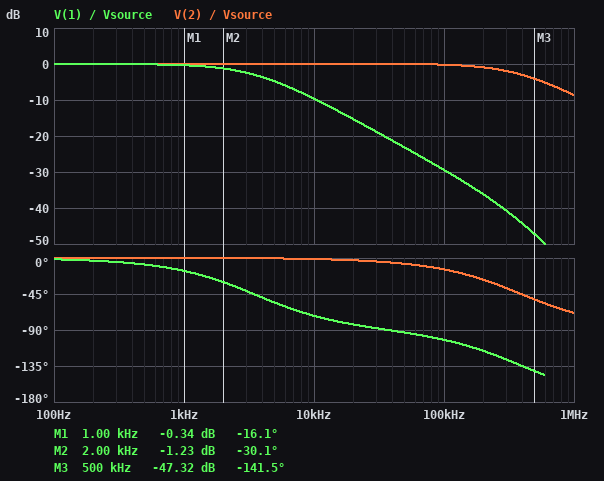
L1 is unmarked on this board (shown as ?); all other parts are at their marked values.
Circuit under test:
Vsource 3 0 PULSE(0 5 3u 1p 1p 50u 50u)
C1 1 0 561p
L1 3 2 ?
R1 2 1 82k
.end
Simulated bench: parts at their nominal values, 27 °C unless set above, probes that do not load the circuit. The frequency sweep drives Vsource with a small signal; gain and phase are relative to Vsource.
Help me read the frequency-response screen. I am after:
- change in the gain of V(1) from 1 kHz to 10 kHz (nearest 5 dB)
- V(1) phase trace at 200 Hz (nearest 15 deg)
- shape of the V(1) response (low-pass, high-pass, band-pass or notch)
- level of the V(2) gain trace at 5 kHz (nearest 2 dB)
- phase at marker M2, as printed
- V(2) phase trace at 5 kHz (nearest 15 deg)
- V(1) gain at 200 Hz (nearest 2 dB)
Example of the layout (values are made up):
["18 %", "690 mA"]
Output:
["-10 dB", "0 deg", "low-pass", "0 dB", "-30.1 deg", "0 deg", "0 dB"]
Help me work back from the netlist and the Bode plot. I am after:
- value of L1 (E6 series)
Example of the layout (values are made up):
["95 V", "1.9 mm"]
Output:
["33 mH"]
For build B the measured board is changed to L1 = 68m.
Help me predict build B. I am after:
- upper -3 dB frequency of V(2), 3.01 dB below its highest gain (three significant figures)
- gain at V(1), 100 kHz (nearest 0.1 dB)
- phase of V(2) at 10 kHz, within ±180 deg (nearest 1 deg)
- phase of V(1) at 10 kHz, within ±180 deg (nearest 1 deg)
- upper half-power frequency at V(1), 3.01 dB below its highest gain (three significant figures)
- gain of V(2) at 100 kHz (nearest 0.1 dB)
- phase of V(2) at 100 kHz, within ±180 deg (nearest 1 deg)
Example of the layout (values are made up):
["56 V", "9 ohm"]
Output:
["190 kHz", "-30.1 dB", "-3 deg", "-74 deg", "3.52 kHz", "-0.9 dB", "-28 deg"]
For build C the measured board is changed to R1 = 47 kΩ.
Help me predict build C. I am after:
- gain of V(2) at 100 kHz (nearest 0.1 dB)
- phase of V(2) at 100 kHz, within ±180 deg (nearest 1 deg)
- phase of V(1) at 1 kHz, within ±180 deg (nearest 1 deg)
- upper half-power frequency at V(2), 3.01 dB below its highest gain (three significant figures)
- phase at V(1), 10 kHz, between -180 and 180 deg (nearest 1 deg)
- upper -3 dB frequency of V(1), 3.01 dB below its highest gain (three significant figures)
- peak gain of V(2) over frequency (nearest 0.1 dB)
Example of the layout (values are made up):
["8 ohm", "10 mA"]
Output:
["-0.6 dB", "-24 deg", "-9 deg", "223 kHz", "-61 deg", "6.20 kHz", "0.2 dB"]
